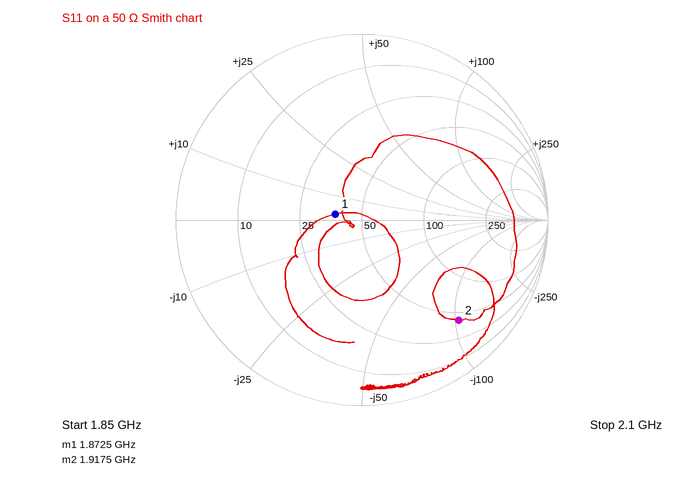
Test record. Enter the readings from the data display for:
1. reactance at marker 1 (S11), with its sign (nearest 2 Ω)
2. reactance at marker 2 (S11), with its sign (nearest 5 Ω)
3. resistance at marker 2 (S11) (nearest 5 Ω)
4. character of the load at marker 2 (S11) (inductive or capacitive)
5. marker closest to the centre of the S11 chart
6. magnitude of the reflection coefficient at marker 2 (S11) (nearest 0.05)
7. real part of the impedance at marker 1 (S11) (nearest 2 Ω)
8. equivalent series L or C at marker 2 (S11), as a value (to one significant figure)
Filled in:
+2 Ω
-105 Ω
40 Ω
capacitive
marker 1
0.75
38 Ω
800 fF
